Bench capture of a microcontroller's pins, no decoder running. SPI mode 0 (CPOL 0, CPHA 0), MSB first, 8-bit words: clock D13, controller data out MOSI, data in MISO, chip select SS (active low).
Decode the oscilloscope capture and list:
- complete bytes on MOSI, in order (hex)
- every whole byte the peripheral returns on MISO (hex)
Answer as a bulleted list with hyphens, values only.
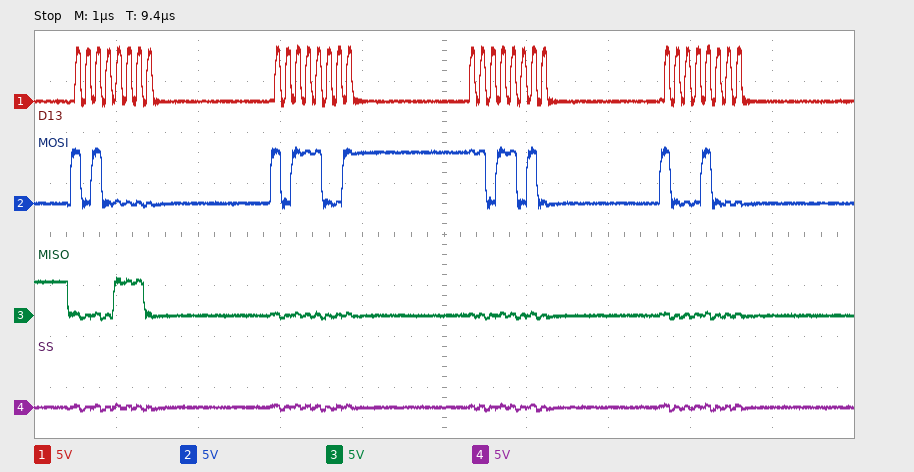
- 0xA0 0xB9 0xDA 0x88
- 0x0E 0x00 0x00 0x00
